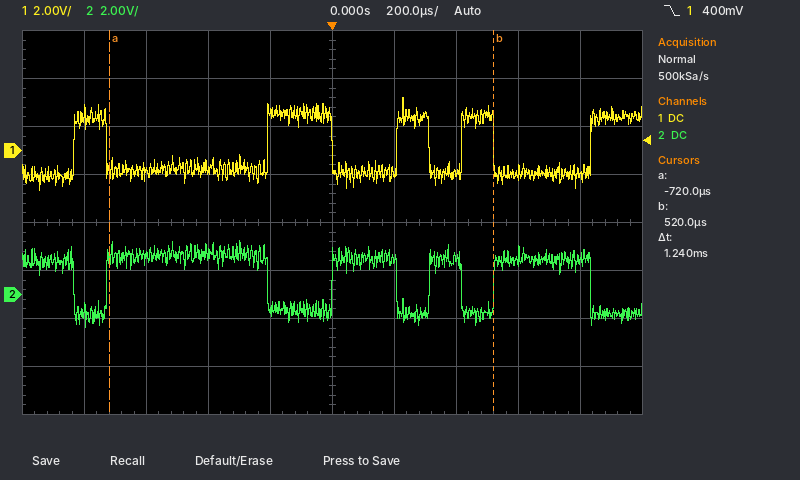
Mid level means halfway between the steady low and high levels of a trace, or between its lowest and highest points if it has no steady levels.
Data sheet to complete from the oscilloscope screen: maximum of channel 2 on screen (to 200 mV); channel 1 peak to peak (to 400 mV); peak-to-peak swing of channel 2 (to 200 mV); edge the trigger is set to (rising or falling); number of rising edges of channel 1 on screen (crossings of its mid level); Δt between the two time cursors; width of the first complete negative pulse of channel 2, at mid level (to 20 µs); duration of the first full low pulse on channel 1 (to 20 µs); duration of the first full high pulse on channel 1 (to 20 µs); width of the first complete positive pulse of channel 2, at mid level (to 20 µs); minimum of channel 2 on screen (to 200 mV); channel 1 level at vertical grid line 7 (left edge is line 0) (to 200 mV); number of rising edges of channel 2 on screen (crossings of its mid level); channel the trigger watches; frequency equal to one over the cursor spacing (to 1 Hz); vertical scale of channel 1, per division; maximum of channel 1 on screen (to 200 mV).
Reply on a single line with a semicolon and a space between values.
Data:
2.2 V; 4.0 V; 3.6 V; falling; 5; 1.24 ms; 100 µs; 520 µs; 100 µs; 520 µs; -1.4 V; -1.0 V; 4; channel 1; 806 Hz; 2 V; 2.2 V
